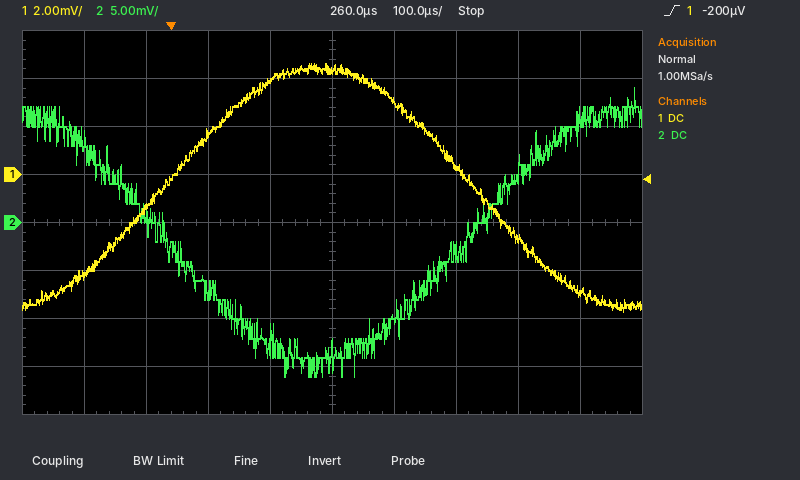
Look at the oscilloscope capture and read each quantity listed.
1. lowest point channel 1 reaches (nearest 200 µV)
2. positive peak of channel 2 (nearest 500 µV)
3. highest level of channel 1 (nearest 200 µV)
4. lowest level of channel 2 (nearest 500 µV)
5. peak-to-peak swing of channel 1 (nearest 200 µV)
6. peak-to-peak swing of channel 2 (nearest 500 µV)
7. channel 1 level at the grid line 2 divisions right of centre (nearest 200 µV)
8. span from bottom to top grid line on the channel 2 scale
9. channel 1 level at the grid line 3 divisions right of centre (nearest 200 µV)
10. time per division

-5.8 mV
14.0 mV
4.6 mV
-16.0 mV
10.4 mV
30.0 mV
400 µV
40 mV
-2.6 mV
100 µs
